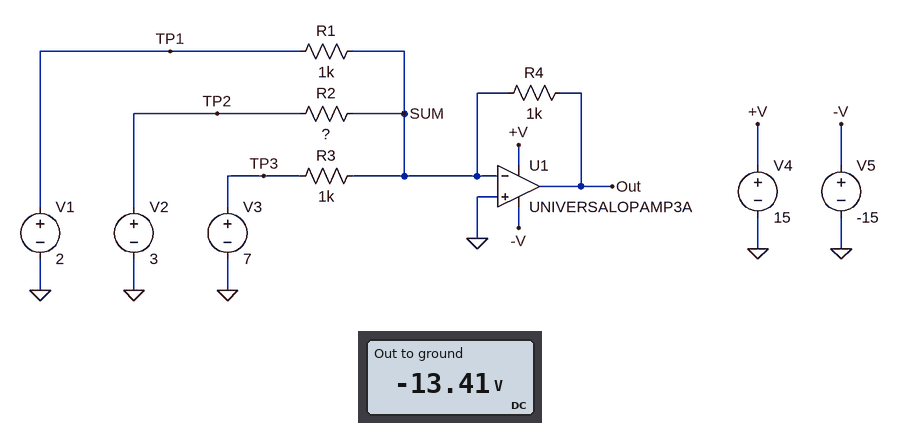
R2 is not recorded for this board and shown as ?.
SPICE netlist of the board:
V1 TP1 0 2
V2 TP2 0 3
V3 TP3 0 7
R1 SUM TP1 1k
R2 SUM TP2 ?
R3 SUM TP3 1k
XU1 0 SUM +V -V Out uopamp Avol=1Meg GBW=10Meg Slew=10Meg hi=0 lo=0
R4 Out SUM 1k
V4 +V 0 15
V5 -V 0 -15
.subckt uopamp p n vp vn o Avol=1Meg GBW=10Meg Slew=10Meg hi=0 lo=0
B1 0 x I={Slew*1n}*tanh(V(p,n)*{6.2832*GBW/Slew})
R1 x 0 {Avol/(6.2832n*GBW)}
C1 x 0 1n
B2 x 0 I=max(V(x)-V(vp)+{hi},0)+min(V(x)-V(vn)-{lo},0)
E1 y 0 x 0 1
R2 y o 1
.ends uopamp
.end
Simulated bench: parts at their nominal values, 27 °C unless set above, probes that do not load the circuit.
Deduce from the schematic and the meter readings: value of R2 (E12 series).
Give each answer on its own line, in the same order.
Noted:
680 Ω
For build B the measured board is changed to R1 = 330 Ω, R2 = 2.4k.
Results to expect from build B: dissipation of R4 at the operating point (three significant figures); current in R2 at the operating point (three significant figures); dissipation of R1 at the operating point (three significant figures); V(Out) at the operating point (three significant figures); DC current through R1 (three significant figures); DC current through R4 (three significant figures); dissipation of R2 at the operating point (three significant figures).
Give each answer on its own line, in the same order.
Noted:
205 mW
1.25 mA
12.1 mW
-14.3 V
6.06 mA
14.3 mA
3.75 mW
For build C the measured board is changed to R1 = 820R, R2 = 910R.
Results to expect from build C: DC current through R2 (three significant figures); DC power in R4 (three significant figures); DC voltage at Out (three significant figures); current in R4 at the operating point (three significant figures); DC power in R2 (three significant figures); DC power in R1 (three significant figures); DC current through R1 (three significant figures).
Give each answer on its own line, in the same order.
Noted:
3.30 mA
162 mW
-12.7 V
12.7 mA
9.89 mW
4.88 mW
2.44 mA
